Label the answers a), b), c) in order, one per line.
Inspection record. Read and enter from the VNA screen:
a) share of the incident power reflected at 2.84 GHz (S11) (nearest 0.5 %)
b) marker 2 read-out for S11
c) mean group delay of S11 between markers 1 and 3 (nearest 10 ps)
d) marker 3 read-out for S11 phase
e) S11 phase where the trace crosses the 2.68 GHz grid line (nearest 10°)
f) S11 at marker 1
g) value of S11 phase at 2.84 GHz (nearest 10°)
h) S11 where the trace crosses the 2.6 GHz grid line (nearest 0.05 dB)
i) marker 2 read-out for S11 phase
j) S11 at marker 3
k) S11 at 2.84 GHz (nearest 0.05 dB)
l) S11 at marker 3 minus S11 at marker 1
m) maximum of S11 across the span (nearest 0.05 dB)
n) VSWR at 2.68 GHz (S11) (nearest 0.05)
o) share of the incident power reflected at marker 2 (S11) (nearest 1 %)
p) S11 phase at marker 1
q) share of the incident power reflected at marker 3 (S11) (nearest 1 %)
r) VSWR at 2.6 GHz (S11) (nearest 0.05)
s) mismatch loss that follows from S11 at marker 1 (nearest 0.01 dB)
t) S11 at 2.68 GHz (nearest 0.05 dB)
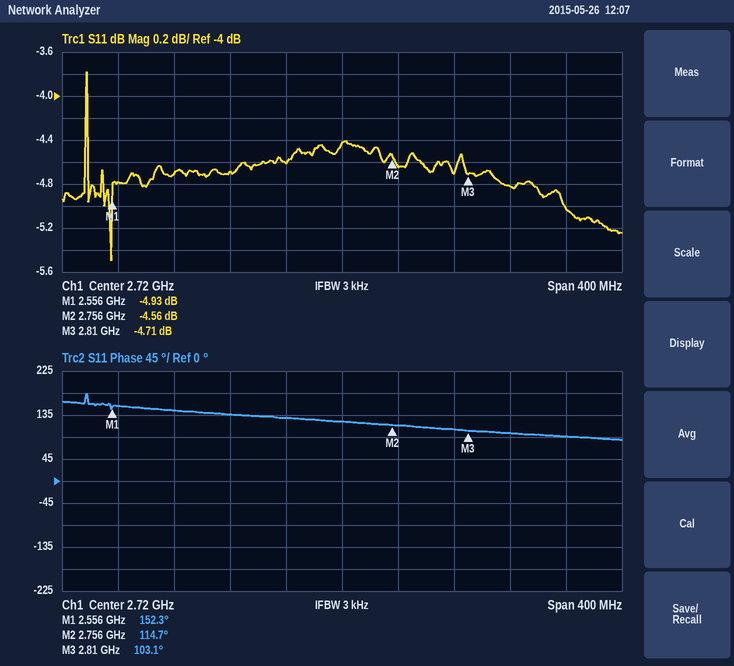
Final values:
a) 33.0 %
b) -4.56 dB
c) 540 ps
d) 103.1°
e) 130°
f) -4.93 dB
g) 100°
h) -4.70 dB
i) 114.7°
j) -4.71 dB
k) -4.80 dB
l) 0.22 dB
m) -3.80 dB
n) 3.85
o) 35 %
p) 152.3°
q) 34 %
r) 3.80
s) 1.68 dB
t) -4.60 dB
